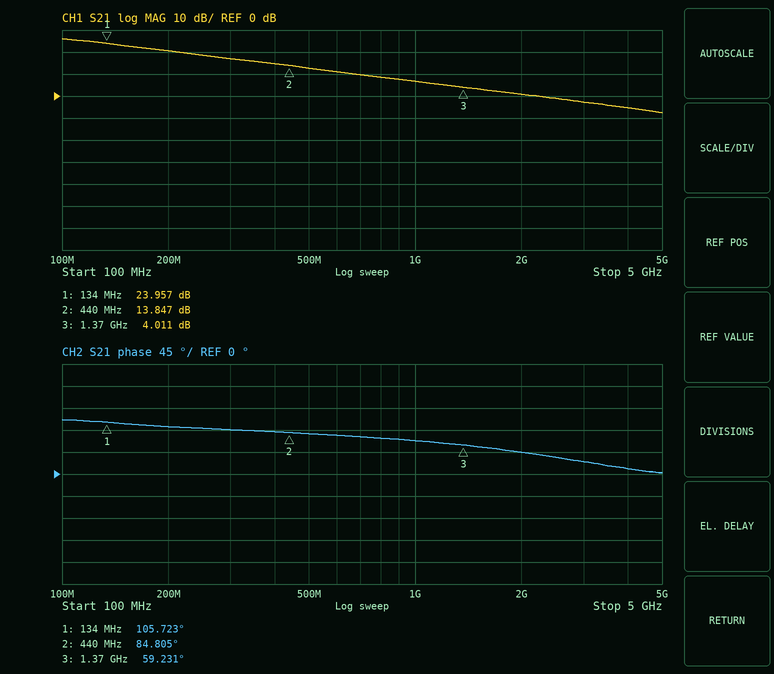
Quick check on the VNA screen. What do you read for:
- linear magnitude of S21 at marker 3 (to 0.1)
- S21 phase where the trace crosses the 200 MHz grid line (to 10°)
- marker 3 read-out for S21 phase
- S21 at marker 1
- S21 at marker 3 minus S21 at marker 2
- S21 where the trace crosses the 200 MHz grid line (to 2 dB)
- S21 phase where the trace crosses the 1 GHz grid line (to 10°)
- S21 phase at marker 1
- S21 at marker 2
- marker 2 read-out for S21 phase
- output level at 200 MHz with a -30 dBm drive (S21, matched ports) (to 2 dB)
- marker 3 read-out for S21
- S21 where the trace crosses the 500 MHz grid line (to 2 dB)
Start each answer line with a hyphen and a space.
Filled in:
- 1.6
- 100°
- 59.231°
- 23.957 dB
- -9.836 dB
- 20 dB
- 70°
- 105.723°
- 13.847 dB
- 84.805°
- -10 dBm
- 4.011 dB
- 12 dB
